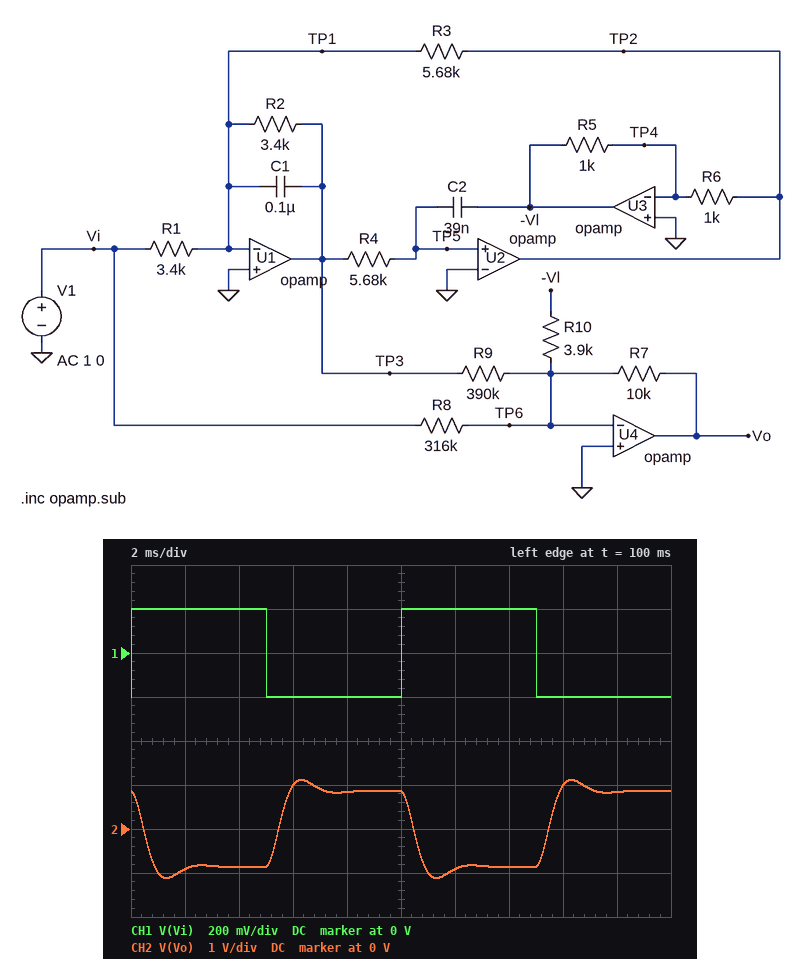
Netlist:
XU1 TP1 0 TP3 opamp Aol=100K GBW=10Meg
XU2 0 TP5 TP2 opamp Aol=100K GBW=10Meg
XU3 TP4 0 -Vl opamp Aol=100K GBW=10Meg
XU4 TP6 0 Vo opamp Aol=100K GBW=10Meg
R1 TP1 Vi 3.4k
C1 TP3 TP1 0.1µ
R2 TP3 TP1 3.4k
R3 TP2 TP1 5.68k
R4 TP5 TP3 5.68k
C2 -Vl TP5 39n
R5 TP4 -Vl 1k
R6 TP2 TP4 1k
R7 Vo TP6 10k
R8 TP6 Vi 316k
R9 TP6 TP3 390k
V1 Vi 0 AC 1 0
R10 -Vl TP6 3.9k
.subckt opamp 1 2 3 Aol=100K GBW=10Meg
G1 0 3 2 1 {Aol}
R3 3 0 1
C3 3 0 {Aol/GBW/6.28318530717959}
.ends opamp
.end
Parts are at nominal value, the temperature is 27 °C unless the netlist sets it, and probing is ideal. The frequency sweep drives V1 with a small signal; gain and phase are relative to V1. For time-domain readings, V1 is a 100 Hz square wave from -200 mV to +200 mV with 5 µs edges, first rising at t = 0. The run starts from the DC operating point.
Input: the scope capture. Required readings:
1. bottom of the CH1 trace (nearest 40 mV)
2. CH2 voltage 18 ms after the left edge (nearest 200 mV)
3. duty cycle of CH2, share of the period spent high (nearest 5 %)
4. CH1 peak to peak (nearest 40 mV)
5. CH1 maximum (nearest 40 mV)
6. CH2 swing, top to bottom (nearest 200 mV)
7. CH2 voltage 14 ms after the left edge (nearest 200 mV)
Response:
-200 mV
800 mV
50 %
400 mV
200 mV
2.2 V
-800 mV
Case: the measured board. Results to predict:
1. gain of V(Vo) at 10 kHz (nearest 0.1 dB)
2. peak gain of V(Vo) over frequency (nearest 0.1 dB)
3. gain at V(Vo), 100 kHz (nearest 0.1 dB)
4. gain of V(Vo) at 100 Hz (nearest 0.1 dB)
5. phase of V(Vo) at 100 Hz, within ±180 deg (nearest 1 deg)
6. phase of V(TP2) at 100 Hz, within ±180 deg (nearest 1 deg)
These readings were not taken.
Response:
-32.8 dB
13.7 dB
-30.0 dB
12.9 dB
166 deg
166 deg
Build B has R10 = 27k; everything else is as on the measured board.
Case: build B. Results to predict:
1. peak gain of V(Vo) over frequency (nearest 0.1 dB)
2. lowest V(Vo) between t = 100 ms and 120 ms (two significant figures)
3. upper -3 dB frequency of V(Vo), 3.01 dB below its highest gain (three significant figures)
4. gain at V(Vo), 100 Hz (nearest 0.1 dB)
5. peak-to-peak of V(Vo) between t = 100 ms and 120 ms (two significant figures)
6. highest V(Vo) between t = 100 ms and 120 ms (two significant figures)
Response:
-2.9 dB
-170 mV
506 Hz
-3.6 dB
330 mV
170 mV
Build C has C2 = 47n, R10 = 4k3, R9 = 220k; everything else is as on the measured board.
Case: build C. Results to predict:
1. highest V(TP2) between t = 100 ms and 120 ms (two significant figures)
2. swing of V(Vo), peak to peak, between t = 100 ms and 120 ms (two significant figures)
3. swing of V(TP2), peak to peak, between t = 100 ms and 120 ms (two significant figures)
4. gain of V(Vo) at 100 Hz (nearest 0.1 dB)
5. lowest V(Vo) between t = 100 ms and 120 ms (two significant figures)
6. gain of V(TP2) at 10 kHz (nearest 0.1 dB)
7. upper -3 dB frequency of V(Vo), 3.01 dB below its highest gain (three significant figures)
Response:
410 mV
1.9 V
820 mV
12.0 dB
-960 mV
-51.1 dB
460 Hz
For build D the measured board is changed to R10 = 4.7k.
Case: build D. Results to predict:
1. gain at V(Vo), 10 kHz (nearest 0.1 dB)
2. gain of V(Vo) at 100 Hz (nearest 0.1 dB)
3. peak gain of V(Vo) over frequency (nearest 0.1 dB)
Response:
-32.2 dB
11.3 dB
12.1 dB
